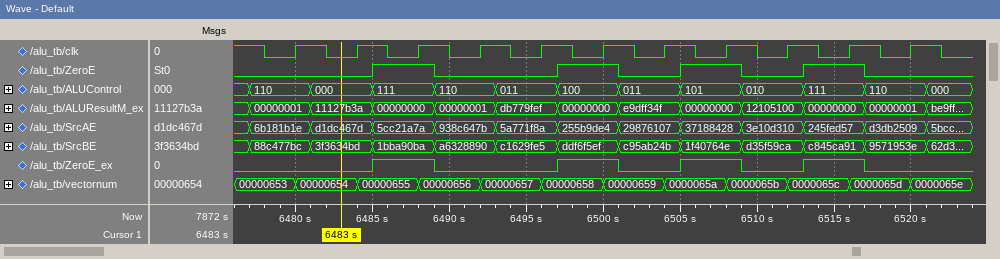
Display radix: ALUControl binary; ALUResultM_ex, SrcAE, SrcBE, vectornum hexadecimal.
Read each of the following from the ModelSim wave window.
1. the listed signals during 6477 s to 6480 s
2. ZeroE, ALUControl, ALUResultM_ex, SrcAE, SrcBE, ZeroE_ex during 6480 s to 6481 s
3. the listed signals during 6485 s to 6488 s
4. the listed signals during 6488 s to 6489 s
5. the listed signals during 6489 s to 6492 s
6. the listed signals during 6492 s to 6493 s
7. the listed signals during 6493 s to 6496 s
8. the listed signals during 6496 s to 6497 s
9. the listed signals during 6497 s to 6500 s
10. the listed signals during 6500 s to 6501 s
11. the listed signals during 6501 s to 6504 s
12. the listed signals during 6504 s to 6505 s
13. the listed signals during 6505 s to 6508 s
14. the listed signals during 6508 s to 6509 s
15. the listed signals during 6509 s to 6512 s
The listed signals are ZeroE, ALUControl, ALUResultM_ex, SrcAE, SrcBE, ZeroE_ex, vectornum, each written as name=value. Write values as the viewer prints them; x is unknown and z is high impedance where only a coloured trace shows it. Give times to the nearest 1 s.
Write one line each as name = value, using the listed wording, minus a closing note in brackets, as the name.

the listed signals during 6477 s to 6480 s = ZeroE=0, ALUControl=110, ALUResultM_ex=00000001, SrcAE=6b181b1e, SrcBE=88c477bc, ZeroE_ex=0, vectornum=00000653
ZeroE, ALUControl, ALUResultM_ex, SrcAE, SrcBE, ZeroE_ex during 6480 s to 6481 s = ZeroE=0, ALUControl=110, ALUResultM_ex=00000001, SrcAE=6b181b1e, SrcBE=88c477bc, ZeroE_ex=0
the listed signals during 6485 s to 6488 s = ZeroE=1, ALUControl=111, ALUResultM_ex=00000000, SrcAE=5cc21a7a, SrcBE=1bba90ba, ZeroE_ex=1, vectornum=00000655
the listed signals during 6488 s to 6489 s = ZeroE=1, ALUControl=111, ALUResultM_ex=00000000, SrcAE=5cc21a7a, SrcBE=1bba90ba, ZeroE_ex=1, vectornum=00000656
the listed signals during 6489 s to 6492 s = ZeroE=0, ALUControl=110, ALUResultM_ex=00000001, SrcAE=938c647b, SrcBE=a6328890, ZeroE_ex=0, vectornum=00000656
the listed signals during 6492 s to 6493 s = ZeroE=0, ALUControl=110, ALUResultM_ex=00000001, SrcAE=938c647b, SrcBE=a6328890, ZeroE_ex=0, vectornum=00000657
the listed signals during 6493 s to 6496 s = ZeroE=0, ALUControl=011, ALUResultM_ex=db779fef, SrcAE=5a771f8a, SrcBE=c1629fe5, ZeroE_ex=0, vectornum=00000657
the listed signals during 6496 s to 6497 s = ZeroE=0, ALUControl=011, ALUResultM_ex=db779fef, SrcAE=5a771f8a, SrcBE=c1629fe5, ZeroE_ex=0, vectornum=00000658
the listed signals during 6497 s to 6500 s = ZeroE=1, ALUControl=100, ALUResultM_ex=00000000, SrcAE=255b9de4, SrcBE=ddf6f5ef, ZeroE_ex=1, vectornum=00000658
the listed signals during 6500 s to 6501 s = ZeroE=1, ALUControl=100, ALUResultM_ex=00000000, SrcAE=255b9de4, SrcBE=ddf6f5ef, ZeroE_ex=1, vectornum=00000659
the listed signals during 6501 s to 6504 s = ZeroE=0, ALUControl=011, ALUResultM_ex=e9dff34f, SrcAE=29876107, SrcBE=c95ab24b, ZeroE_ex=0, vectornum=00000659
the listed signals during 6504 s to 6505 s = ZeroE=0, ALUControl=011, ALUResultM_ex=e9dff34f, SrcAE=29876107, SrcBE=c95ab24b, ZeroE_ex=0, vectornum=0000065a
the listed signals during 6505 s to 6508 s = ZeroE=1, ALUControl=101, ALUResultM_ex=00000000, SrcAE=37188428, SrcBE=1f40764e, ZeroE_ex=1, vectornum=0000065a
the listed signals during 6508 s to 6509 s = ZeroE=1, ALUControl=101, ALUResultM_ex=00000000, SrcAE=37188428, SrcBE=1f40764e, ZeroE_ex=1, vectornum=0000065b
the listed signals during 6509 s to 6512 s = ZeroE=0, ALUControl=010, ALUResultM_ex=12105100, SrcAE=3e10d310, SrcBE=d35f59ca, ZeroE_ex=0, vectornum=0000065b
